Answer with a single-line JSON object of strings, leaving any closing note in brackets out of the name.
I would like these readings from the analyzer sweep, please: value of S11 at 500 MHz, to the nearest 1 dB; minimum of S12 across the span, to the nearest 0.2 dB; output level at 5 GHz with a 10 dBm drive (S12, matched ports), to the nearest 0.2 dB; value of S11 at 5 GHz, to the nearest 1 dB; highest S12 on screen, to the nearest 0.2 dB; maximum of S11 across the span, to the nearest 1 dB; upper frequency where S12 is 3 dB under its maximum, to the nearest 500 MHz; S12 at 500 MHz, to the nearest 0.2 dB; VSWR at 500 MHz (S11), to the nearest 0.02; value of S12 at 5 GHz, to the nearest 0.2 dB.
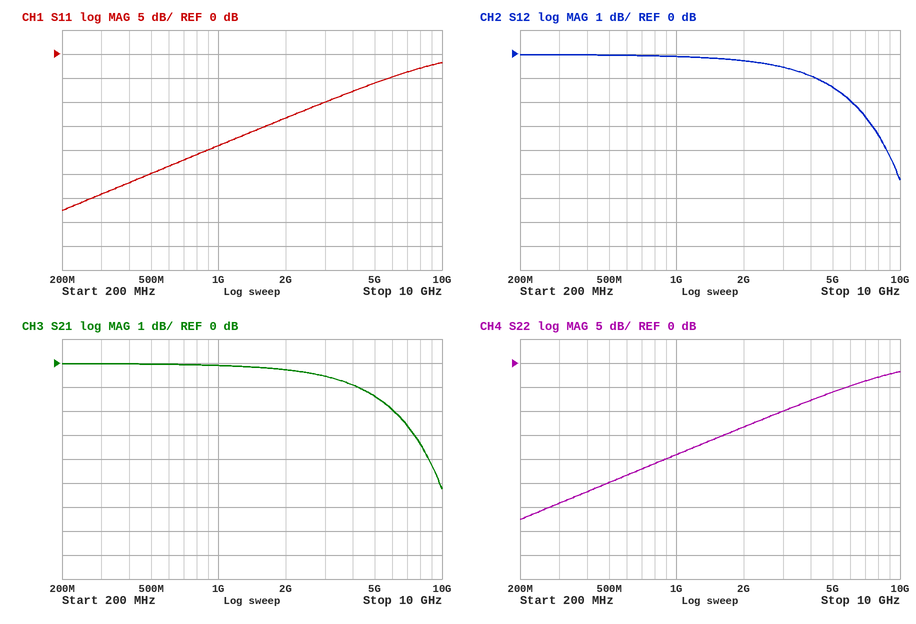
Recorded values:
{"value of S11 at 500 MHz, to the nearest 1 dB": "-25 dB", "minimum of S12 across the span, to the nearest 0.2 dB": "-5.2 dB", "output level at 5 GHz with a 10 dBm drive (S12, matched ports), to the nearest 0.2 dB": "8.6 dBm", "value of S11 at 5 GHz, to the nearest 1 dB": "-6 dB", "highest S12 on screen, to the nearest 0.2 dB": "0.0 dB", "maximum of S11 across the span, to the nearest 1 dB": "-2 dB", "upper frequency where S12 is 3 dB under its maximum, to the nearest 500 MHz": "7.5 GHz", "S12 at 500 MHz, to the nearest 0.2 dB": "0.0 dB", "VSWR at 500 MHz (S11), to the nearest 0.02": "1.12", "value of S12 at 5 GHz, to the nearest 0.2 dB": "-1.4 dB"}
